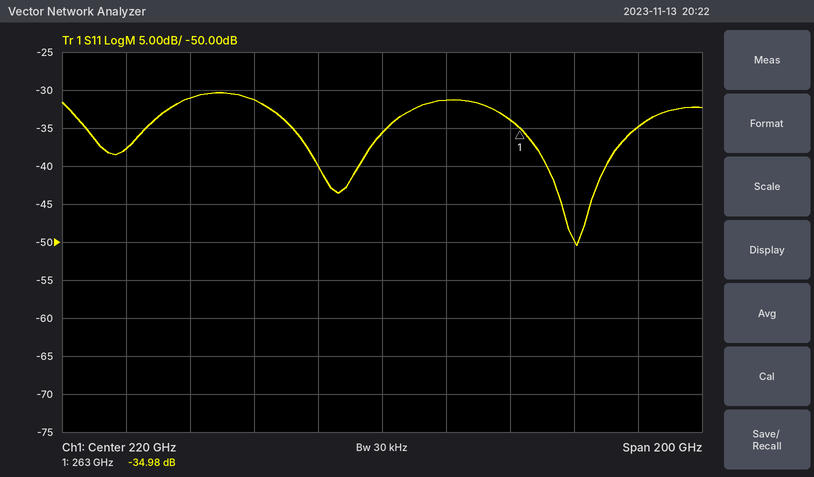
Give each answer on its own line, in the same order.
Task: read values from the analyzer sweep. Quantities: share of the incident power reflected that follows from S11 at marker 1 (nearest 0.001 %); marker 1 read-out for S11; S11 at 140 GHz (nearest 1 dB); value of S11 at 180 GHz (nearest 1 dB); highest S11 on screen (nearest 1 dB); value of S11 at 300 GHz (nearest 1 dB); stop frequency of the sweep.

0.032 %
-34.98 dB
-38 dB
-31 dB
-30 dB
-35 dB
320 GHz
